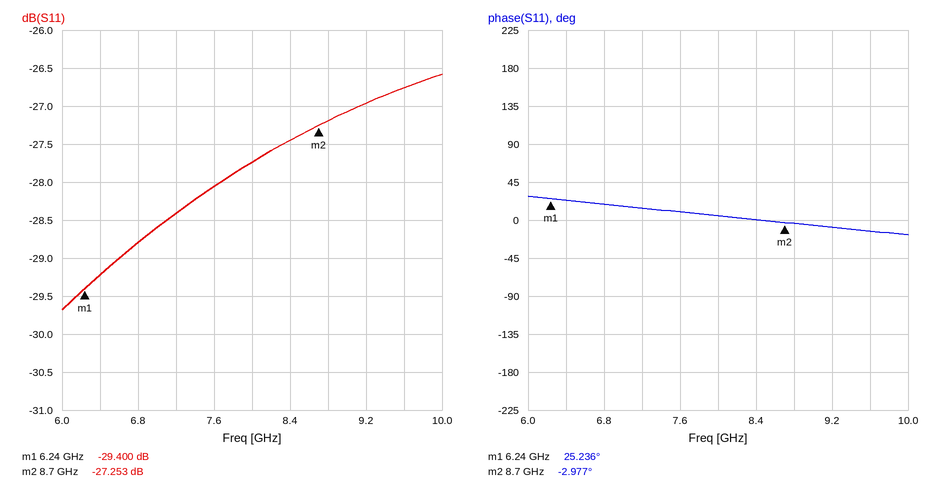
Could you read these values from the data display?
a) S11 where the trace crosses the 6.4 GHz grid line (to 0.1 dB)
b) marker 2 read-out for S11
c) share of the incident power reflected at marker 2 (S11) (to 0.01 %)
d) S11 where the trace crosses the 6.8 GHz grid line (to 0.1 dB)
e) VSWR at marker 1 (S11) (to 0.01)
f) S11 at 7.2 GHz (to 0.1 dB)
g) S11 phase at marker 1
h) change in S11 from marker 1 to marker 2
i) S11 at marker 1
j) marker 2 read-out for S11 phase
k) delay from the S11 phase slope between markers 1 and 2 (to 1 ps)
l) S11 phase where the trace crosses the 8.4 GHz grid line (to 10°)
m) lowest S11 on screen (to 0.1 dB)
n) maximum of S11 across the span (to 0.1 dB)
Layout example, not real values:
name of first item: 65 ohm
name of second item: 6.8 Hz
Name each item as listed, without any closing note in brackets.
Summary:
S11 where the trace crosses the 6.4 GHz grid line: -29.2 dB
marker 2 read-out for S11: -27.253 dB
share of the incident power reflected at marker 2 (S11): 0.19 %
S11 where the trace crosses the 6.8 GHz grid line: -28.8 dB
VSWR at marker 1 (S11): 1.07
S11 at 7.2 GHz: -28.4 dB
S11 phase at marker 1: 25.236°
change in S11 from marker 1 to marker 2: 2.147 dB
S11 at marker 1: -29.400 dB
marker 2 read-out for S11 phase: -2.977°
delay from the S11 phase slope between markers 1 and 2: 32 ps
S11 phase where the trace crosses the 8.4 GHz grid line: 0°
lowest S11 on screen: -29.7 dB
maximum of S11 across the span: -26.6 dB
